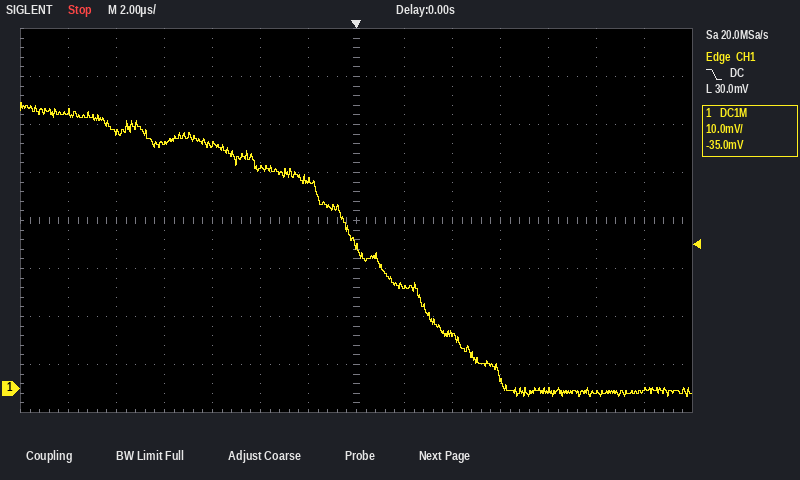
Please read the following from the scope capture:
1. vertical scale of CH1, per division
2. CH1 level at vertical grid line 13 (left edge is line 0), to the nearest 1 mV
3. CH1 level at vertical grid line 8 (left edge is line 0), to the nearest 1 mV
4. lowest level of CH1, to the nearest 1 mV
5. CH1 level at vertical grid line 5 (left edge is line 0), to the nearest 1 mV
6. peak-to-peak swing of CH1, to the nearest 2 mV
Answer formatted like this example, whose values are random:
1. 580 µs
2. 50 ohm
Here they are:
1. 10 mV
2. 0 mV
3. 21 mV
4. -2 mV
5. 46 mV
6. 62 mV
